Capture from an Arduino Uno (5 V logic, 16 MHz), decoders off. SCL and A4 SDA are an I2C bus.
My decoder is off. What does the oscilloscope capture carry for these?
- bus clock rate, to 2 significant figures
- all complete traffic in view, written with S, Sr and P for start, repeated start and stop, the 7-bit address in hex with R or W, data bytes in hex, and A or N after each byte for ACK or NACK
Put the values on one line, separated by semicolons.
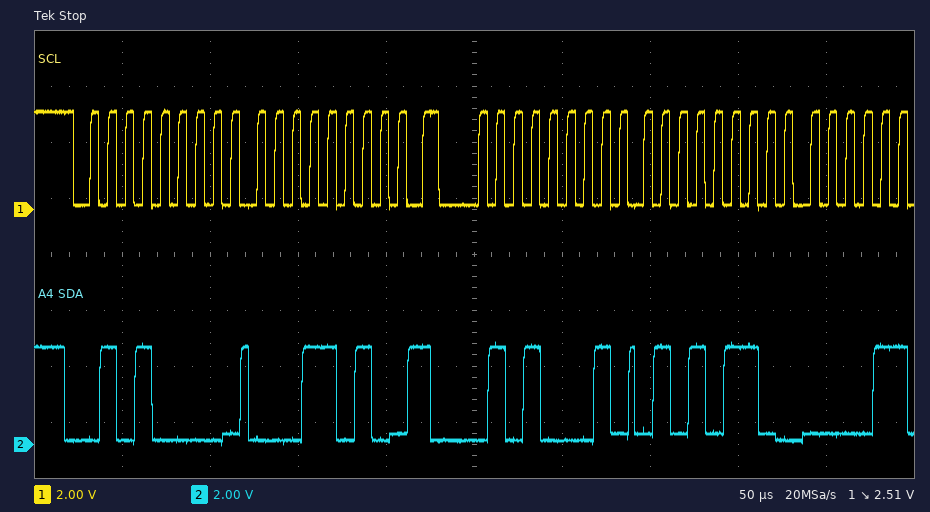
100 kHz; S 28W A 1A A Sr 28R A 56 A
